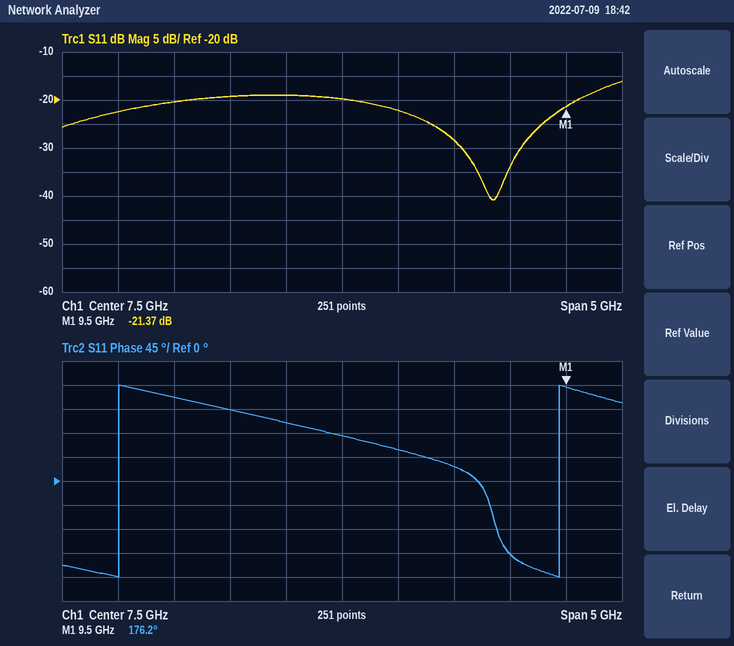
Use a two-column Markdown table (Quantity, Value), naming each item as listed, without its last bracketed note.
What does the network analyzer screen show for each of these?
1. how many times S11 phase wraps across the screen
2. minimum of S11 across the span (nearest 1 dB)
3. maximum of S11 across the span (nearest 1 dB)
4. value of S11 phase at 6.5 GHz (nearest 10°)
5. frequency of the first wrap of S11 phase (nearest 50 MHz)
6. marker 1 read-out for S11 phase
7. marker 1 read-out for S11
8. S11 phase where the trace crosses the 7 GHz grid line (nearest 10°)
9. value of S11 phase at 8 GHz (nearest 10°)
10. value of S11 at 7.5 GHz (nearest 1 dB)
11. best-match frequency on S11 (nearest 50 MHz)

| Quantity | Value |
|---|---|
| how many times S11 phase wraps across the screen | 2 |
| minimum of S11 across the span | -41 dB |
| maximum of S11 across the span | -16 dB |
| value of S11 phase at 6.5 GHz | 130° |
| frequency of the first wrap of S11 phase | 5.50 GHz |
| marker 1 read-out for S11 phase | 176.2° |
| marker 1 read-out for S11 | -21.37 dB |
| S11 phase where the trace crosses the 7 GHz grid line | 110° |
| value of S11 phase at 8 GHz | 60° |
| value of S11 at 7.5 GHz | -20 dB |
| best-match frequency on S11 | 8.85 GHz |
